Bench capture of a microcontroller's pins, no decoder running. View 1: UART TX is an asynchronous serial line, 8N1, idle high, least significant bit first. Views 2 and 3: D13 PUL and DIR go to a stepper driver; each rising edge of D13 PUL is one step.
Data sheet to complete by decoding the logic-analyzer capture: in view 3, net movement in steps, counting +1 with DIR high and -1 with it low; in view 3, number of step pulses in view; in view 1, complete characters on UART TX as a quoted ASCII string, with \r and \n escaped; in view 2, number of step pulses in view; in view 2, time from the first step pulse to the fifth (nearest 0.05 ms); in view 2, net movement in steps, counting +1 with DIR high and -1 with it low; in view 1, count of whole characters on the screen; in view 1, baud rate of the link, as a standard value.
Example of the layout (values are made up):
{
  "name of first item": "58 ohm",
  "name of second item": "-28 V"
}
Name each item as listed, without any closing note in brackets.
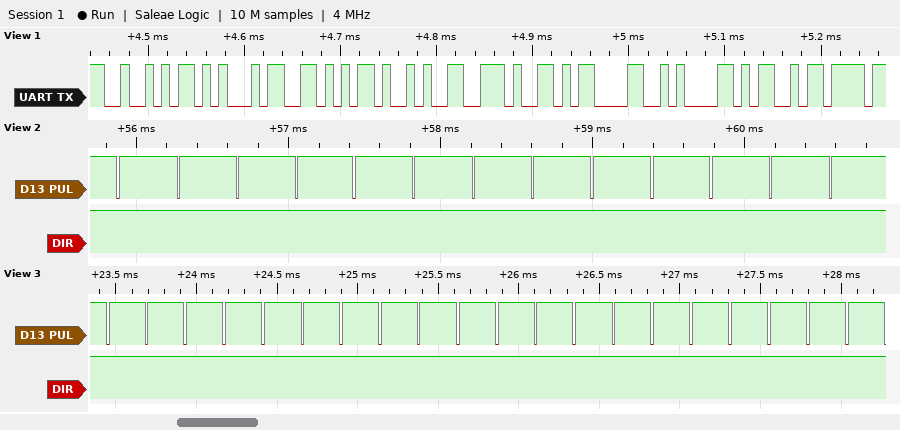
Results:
{
  "in view 3, net movement in steps, counting +1 with DIR high and -1 with it low": "+20",
  "in view 3, number of step pulses in view": "20",
  "in view 1, complete characters on UART TX as a quoted ASCII string, with \\r and \\n escaped": "\"REV).\\r\\nM\"",
  "in view 2, number of step pulses in view": "13",
  "in view 2, time from the first step pulse to the fifth": "1.55 ms",
  "in view 2, net movement in steps, counting +1 with DIR high and -1 with it low": "+13",
  "in view 1, count of whole characters on the screen": "8",
  "in view 1, baud rate of the link, as a standard value": "115200 baud"
}
